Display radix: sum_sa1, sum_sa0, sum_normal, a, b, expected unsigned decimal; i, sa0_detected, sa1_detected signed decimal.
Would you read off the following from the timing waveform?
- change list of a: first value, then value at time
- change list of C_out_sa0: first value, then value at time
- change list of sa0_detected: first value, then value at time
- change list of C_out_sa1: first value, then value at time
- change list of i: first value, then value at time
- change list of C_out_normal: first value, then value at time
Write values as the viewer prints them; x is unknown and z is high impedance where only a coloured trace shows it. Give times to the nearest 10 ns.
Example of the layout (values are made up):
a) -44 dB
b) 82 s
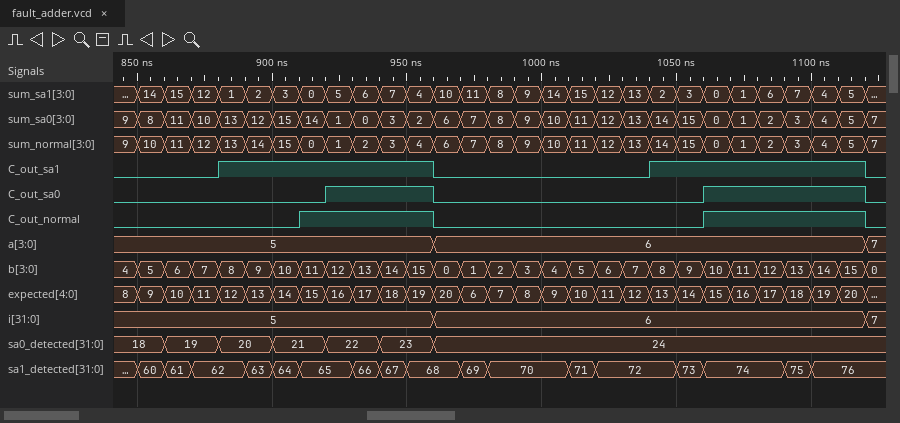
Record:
a) 5, 6 at 960 ns, 7 at 1120 ns
b) 0, 1 at 920 ns, 0 at 960 ns, 1 at 1060 ns, 0 at 1120 ns
c) 18, 19 at 860 ns, 20 at 880 ns, 21 at 900 ns, 22 at 920 ns, 23 at 940 ns, 24 at 960 ns
d) 0, 1 at 880 ns, 0 at 960 ns, 1 at 1040 ns, 0 at 1120 ns
e) 5, 6 at 960 ns, 7 at 1120 ns
f) 0, 1 at 910 ns, 0 at 960 ns, 1 at 1060 ns, 0 at 1120 ns
